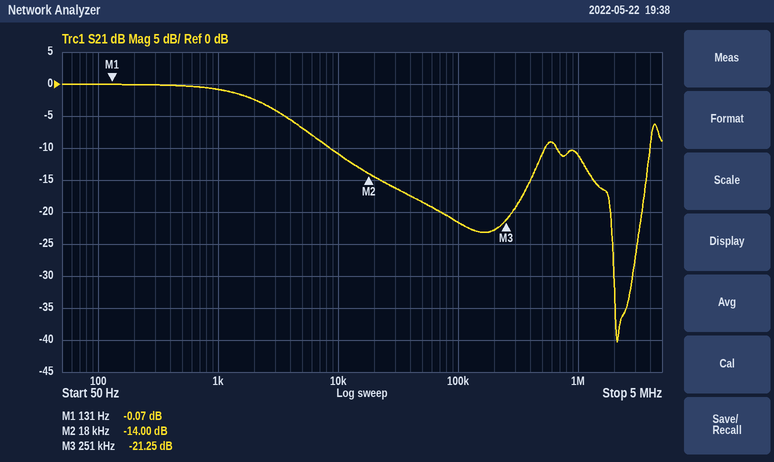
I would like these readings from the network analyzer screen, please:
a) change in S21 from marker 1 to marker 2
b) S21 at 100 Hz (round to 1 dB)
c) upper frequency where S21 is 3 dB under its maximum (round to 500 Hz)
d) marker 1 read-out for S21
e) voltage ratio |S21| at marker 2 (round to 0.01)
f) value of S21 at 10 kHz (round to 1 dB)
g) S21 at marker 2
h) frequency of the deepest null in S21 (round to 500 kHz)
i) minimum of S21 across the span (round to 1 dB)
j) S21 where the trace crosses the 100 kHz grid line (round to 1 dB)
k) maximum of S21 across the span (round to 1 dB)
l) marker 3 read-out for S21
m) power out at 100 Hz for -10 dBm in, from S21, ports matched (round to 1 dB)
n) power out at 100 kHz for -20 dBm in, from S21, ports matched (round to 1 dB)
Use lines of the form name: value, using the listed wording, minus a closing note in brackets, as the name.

change in S21 from marker 1 to marker 2: -13.93 dB
S21 at 100 Hz: 0 dB
upper frequency where S21 is 3 dB under its maximum: 2.5 kHz
marker 1 read-out for S21: -0.07 dB
voltage ratio |S21| at marker 2: 0.20
value of S21 at 10 kHz: -11 dB
S21 at marker 2: -14.00 dB
frequency of the deepest null in S21: 2.0 MHz
minimum of S21 across the span: -40 dB
S21 where the trace crosses the 100 kHz grid line: -22 dB
maximum of S21 across the span: 0 dB
marker 3 read-out for S21: -21.25 dB
power out at 100 Hz for -10 dBm in, from S21, ports matched: -10 dBm
power out at 100 kHz for -20 dBm in, from S21, ports matched: -42 dBm
